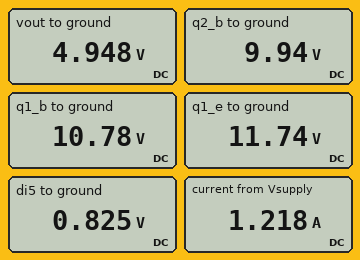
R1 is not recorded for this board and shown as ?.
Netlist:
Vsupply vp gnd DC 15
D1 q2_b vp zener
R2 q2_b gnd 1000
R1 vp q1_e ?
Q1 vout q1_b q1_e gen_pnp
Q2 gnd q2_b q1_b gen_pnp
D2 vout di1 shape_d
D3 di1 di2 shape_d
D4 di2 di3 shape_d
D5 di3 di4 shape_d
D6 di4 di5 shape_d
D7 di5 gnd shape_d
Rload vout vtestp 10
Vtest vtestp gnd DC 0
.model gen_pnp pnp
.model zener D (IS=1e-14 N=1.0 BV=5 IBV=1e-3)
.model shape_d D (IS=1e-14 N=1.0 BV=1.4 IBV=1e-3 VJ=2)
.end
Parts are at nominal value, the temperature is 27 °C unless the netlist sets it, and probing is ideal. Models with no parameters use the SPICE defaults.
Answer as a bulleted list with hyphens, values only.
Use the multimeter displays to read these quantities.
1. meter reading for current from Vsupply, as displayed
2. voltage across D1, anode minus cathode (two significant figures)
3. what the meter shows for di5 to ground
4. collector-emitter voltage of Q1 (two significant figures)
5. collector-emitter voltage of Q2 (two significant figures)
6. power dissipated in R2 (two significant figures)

- 1.218 A
- -5.1 V
- 0.825 V
- -6.8 V
- -11 V
- 99 mW
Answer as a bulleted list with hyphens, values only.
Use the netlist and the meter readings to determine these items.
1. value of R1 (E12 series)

- 2.7 Ω
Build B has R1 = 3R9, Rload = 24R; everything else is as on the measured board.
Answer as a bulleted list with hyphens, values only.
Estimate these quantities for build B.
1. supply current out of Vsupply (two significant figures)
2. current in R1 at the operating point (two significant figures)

- 850 mA
- 840 mA
